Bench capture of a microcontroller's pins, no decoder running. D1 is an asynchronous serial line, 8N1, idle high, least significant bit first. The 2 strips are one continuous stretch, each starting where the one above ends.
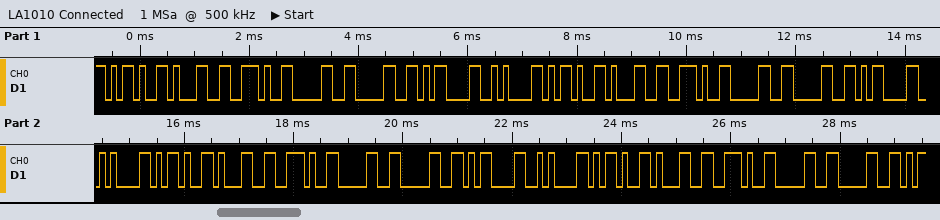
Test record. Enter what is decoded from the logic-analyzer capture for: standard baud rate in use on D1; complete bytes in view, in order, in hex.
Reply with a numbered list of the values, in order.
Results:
1. 9600 baud
2. 2D 31 2E 30 30 0D 0A 2D 31 2E 30 30 0D 0A 2D 31 2E 30 30 0D 0A 2D 31 2E 30 30
